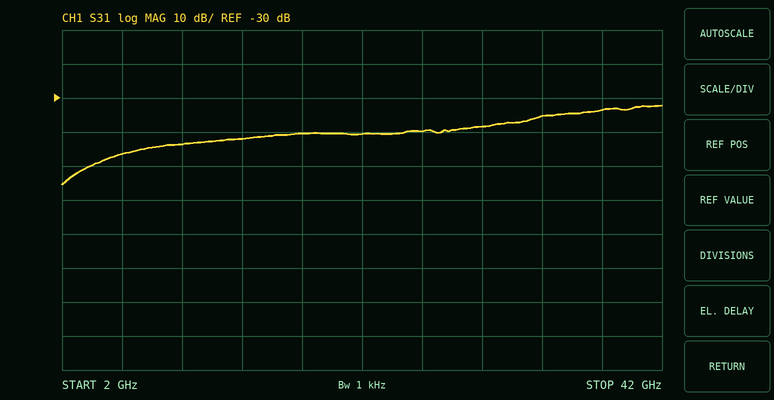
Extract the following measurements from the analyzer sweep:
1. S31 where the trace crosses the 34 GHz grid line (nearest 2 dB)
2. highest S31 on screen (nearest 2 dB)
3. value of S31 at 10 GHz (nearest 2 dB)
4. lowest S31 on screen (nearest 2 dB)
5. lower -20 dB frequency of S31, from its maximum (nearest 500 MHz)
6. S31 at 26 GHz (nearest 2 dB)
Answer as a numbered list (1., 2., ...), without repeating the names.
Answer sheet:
1. -36 dB
2. -32 dB
3. -44 dB
4. -56 dB
5. 3.0 GHz
6. -40 dB
